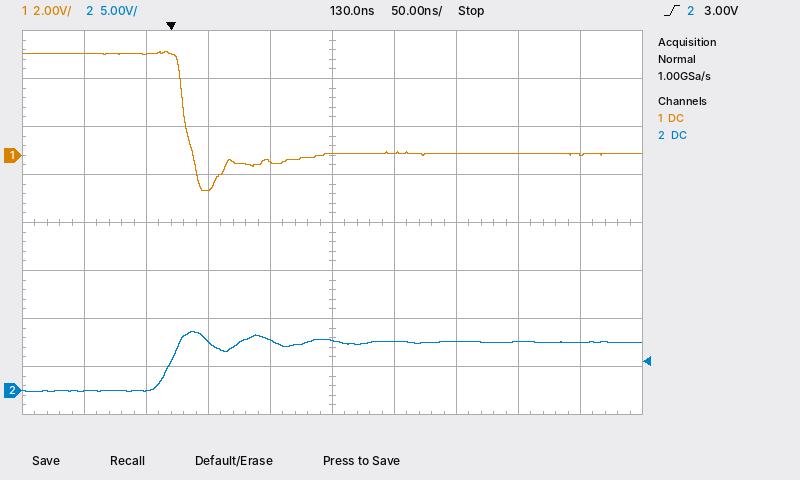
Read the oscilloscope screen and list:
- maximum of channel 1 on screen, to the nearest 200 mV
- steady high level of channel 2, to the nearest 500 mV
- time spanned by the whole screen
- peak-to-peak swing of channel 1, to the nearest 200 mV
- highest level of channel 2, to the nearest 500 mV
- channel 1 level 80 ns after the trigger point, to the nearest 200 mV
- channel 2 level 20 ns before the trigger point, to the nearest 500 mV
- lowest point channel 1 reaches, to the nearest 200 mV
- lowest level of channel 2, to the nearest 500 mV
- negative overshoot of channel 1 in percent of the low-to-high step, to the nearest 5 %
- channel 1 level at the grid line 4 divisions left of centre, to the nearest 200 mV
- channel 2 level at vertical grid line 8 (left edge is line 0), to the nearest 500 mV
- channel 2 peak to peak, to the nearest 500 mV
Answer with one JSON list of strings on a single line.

["4.4 V", "5.0 V", "500 ns", "5.8 V", "6.0 V", "-200 mV", "0.0 V", "-1.4 V", "0.0 V", "35 %", "4.2 V", "5.0 V", "6.0 V"]
